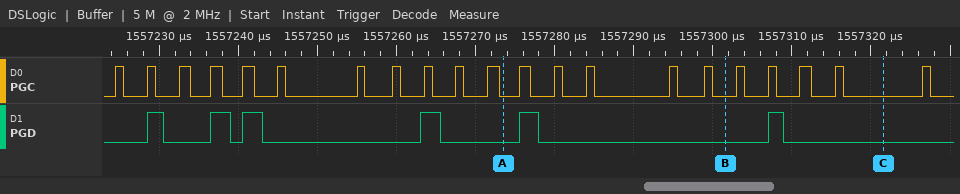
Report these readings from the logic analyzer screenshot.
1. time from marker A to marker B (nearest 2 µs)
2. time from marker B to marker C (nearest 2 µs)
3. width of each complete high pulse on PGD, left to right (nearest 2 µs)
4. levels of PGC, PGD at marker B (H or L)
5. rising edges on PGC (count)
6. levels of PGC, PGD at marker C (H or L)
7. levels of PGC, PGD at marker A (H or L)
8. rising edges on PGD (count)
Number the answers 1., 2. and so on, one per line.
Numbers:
1. 28 µs
2. 20 µs
3. 2 µs, 2 µs, 2 µs, 2 µs, 2 µs, 2 µs
4. PGC=L, PGD=L
5. 21
6. PGC=L, PGD=L
7. PGC=L, PGD=L
8. 6
